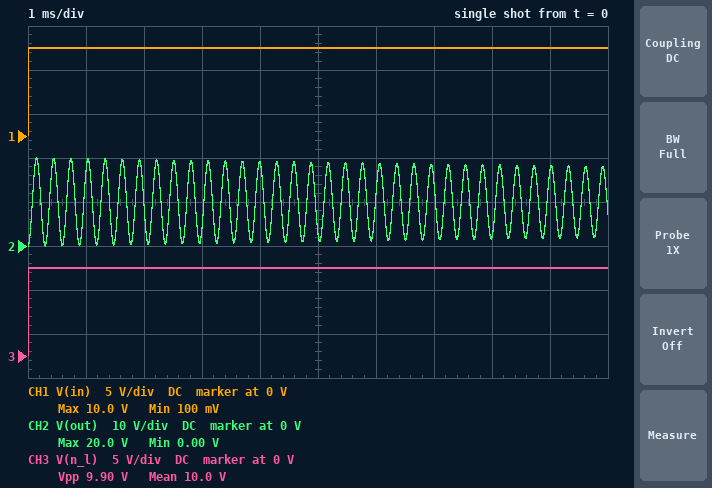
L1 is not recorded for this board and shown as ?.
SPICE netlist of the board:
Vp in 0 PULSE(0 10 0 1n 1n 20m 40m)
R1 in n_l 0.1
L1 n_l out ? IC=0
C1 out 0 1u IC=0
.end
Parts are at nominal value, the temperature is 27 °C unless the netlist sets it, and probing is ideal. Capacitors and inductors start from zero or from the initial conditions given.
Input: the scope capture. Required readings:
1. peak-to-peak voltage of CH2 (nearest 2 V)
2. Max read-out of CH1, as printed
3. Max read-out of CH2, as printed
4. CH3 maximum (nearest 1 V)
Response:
20 V
10.0 V
20.0 V
10 V
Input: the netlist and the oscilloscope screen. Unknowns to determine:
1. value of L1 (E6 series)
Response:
2.2 mH
